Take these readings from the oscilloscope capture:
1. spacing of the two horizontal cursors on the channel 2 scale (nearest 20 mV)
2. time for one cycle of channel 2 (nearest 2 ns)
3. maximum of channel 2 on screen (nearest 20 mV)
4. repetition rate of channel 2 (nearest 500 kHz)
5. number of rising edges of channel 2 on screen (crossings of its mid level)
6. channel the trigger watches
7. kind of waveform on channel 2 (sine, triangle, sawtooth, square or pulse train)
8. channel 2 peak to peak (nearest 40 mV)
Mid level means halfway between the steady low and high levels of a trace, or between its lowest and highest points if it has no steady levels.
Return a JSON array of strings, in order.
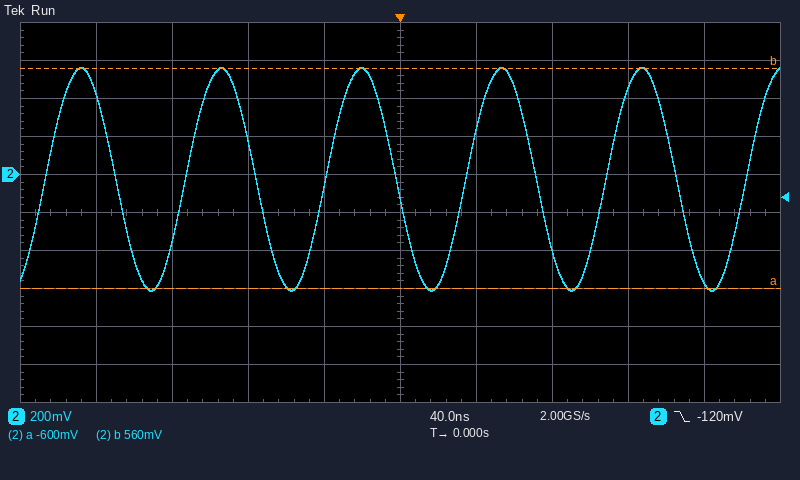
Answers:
["1.16 V", "74 ns", "560 mV", "13.5 MHz", "6", "channel 2", "sine", "1.16 V"]
